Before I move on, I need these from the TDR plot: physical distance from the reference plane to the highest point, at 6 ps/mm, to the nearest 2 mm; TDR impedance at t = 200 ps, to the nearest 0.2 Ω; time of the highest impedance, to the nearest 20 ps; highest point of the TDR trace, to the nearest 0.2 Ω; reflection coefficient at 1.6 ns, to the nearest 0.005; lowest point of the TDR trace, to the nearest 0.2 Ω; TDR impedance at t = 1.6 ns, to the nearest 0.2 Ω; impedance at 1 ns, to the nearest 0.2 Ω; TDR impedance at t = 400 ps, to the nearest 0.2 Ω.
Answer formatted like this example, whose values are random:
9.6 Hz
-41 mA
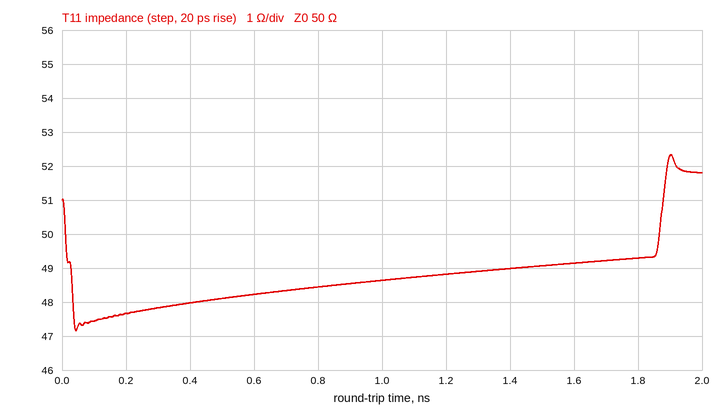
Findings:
158 mm
47.6 Ω
1.90 ns
52.4 Ω
-0.010
47.2 Ω
49.2 Ω
48.6 Ω
48.0 Ω
